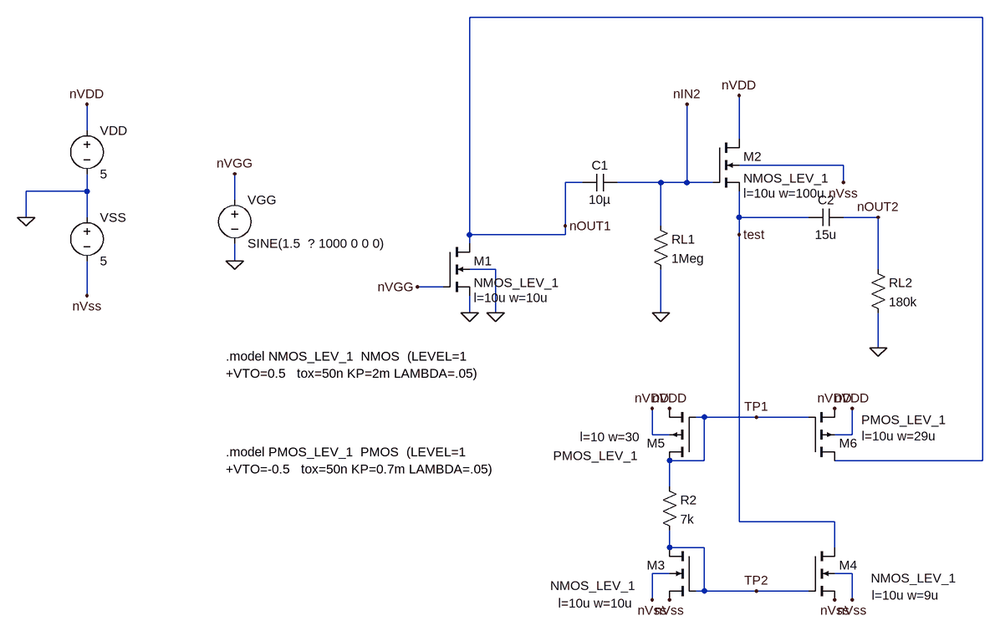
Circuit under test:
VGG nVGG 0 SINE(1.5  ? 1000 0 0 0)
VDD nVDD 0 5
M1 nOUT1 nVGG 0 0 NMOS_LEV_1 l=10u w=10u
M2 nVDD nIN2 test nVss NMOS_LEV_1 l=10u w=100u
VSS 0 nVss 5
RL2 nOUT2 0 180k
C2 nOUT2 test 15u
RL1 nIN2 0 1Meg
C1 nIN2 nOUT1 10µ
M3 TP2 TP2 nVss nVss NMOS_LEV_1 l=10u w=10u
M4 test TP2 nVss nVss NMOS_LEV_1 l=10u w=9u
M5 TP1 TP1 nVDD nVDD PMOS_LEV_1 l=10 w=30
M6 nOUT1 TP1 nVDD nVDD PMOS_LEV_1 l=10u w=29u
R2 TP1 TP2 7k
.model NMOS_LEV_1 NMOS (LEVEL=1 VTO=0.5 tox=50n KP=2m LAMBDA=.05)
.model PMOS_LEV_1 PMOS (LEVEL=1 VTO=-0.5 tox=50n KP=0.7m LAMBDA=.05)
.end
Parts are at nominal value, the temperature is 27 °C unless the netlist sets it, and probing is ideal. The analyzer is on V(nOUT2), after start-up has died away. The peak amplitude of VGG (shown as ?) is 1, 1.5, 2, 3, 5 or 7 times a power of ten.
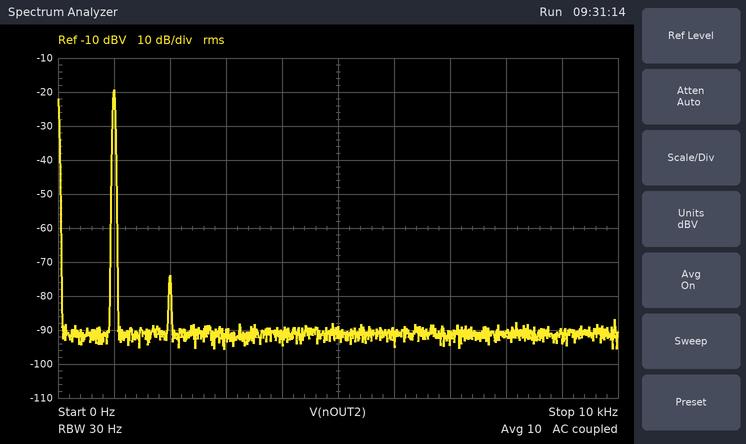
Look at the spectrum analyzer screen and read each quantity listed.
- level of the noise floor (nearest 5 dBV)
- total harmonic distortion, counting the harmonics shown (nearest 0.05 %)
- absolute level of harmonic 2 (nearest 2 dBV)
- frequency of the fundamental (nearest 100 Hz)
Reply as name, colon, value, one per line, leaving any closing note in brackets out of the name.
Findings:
level of the noise floor: -90 dBV
total harmonic distortion, counting the harmonics shown: 0.20 %
absolute level of harmonic 2: -74 dBV
frequency of the fundamental: 1.0 kHz
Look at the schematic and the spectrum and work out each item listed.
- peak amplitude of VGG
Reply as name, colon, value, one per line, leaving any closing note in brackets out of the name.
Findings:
peak amplitude of VGG: 7 mV
